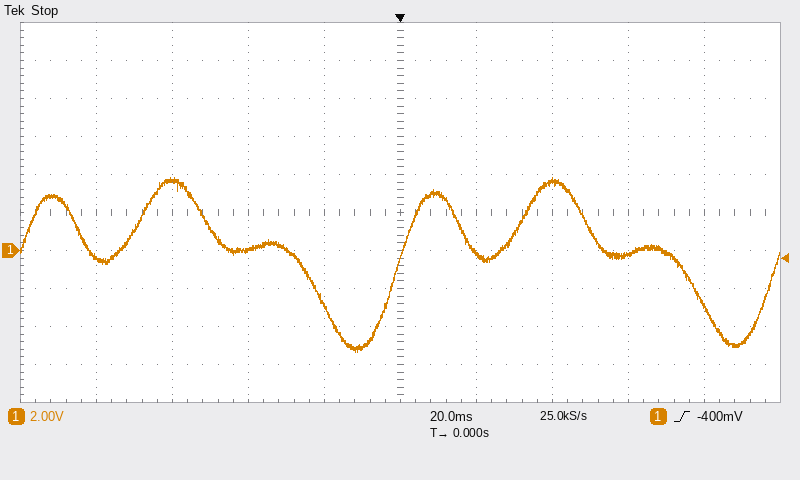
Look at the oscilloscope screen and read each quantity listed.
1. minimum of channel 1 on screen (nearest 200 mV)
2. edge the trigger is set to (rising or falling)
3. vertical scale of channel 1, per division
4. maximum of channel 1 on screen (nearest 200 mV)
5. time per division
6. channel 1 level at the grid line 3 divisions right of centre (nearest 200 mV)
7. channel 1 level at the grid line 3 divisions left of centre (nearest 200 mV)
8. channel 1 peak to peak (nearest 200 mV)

-5.4 V
rising
2 V
3.8 V
20 ms
-200 mV
3.6 V
9.2 V
